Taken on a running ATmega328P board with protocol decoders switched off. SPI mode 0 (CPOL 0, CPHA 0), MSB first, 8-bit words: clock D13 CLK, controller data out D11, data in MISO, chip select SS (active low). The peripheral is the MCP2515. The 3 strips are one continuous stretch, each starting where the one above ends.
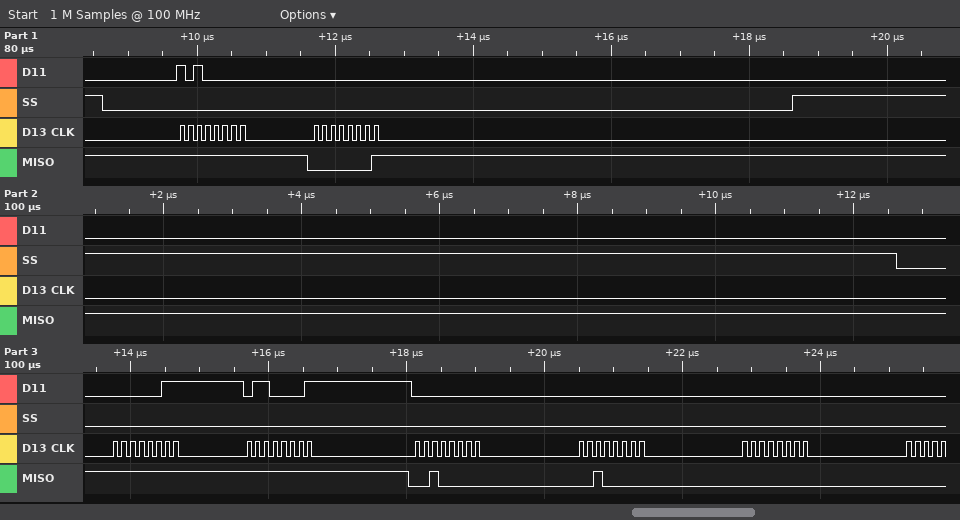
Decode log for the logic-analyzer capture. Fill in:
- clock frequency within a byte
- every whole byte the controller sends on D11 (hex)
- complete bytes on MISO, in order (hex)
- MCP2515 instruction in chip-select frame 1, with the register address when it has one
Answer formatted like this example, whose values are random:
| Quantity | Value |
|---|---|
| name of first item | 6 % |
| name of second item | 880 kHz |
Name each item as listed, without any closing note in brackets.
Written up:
| Quantity | Value |
|---|---|
| clock frequency within a byte | 8 MHz |
| every whole byte the controller sends on D11 | A0 00 03 61 00 00 00 |
| complete bytes on MISO, in order | FF 01 FF FF 20 20 00 |
| MCP2515 instruction in chip-select frame 1, with the register address when it has one | READ STATUS |
